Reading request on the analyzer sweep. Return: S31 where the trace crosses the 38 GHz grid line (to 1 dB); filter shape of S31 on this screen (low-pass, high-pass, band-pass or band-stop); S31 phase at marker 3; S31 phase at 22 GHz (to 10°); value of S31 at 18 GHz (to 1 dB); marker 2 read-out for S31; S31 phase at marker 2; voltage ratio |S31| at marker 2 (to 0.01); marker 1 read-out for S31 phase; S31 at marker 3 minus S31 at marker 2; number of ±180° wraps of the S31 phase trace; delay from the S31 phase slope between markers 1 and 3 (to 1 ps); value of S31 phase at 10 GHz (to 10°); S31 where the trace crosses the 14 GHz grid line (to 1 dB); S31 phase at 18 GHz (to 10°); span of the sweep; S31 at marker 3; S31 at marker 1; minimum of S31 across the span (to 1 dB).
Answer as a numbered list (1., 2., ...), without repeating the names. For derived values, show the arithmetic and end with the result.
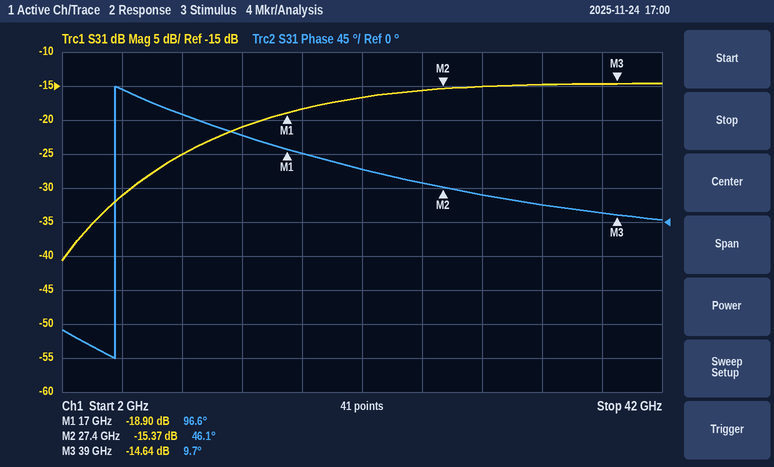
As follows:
1. -15 dB
2. high-pass
3. 9.7°
4. 70°
5. -18 dB
6. -15.37 dB
7. 46.1°
8. 10^(-15.37/20) ≈ 0.17
9. 96.6°
10. -14.64 − (-15.37) = 0.73 dB
11. 1
12. −(9.7° − (96.6°))/(360° × 22 GHz) ≈ 11 ps
13. 140°
14. -21 dB
15. 90°
16. 40 GHz
17. -14.64 dB
18. -18.90 dB
19. -41 dB
